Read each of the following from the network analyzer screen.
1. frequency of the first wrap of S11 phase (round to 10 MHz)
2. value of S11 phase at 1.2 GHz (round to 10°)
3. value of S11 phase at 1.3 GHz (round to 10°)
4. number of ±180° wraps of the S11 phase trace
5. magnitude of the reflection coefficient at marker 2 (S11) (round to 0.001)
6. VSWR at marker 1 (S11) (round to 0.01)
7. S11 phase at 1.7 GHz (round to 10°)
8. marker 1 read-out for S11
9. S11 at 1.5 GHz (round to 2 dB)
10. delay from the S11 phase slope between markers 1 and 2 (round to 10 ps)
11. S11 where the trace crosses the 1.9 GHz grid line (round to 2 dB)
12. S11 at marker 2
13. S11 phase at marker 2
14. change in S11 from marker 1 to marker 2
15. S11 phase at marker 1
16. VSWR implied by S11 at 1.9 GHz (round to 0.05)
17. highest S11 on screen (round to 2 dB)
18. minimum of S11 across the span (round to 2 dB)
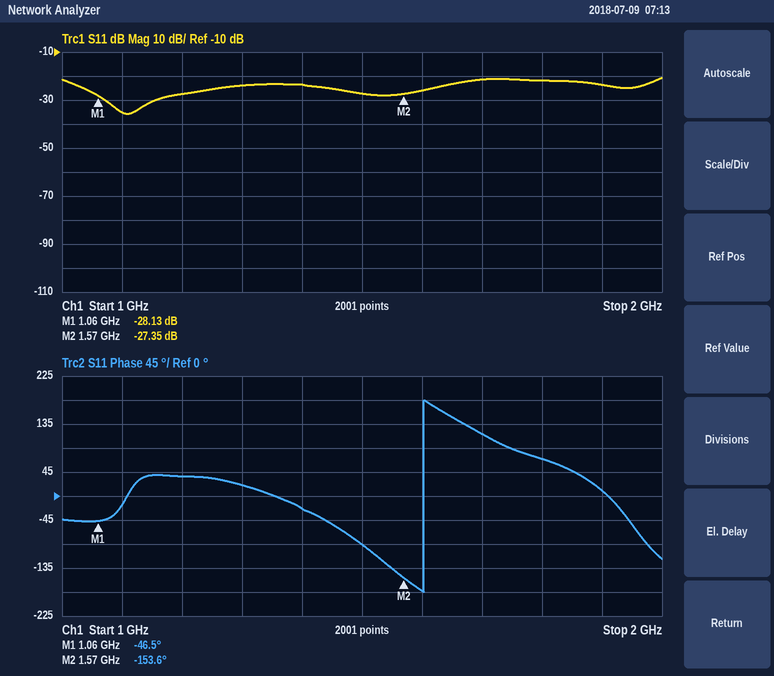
1.60 GHz
40°
20°
1
0.043
1.08
120°
-28.13 dB
-28 dB
580 ps
-24 dB
-27.35 dB
-153.6°
0.78 dB
-46.5°
1.15
-20 dB
-36 dB
